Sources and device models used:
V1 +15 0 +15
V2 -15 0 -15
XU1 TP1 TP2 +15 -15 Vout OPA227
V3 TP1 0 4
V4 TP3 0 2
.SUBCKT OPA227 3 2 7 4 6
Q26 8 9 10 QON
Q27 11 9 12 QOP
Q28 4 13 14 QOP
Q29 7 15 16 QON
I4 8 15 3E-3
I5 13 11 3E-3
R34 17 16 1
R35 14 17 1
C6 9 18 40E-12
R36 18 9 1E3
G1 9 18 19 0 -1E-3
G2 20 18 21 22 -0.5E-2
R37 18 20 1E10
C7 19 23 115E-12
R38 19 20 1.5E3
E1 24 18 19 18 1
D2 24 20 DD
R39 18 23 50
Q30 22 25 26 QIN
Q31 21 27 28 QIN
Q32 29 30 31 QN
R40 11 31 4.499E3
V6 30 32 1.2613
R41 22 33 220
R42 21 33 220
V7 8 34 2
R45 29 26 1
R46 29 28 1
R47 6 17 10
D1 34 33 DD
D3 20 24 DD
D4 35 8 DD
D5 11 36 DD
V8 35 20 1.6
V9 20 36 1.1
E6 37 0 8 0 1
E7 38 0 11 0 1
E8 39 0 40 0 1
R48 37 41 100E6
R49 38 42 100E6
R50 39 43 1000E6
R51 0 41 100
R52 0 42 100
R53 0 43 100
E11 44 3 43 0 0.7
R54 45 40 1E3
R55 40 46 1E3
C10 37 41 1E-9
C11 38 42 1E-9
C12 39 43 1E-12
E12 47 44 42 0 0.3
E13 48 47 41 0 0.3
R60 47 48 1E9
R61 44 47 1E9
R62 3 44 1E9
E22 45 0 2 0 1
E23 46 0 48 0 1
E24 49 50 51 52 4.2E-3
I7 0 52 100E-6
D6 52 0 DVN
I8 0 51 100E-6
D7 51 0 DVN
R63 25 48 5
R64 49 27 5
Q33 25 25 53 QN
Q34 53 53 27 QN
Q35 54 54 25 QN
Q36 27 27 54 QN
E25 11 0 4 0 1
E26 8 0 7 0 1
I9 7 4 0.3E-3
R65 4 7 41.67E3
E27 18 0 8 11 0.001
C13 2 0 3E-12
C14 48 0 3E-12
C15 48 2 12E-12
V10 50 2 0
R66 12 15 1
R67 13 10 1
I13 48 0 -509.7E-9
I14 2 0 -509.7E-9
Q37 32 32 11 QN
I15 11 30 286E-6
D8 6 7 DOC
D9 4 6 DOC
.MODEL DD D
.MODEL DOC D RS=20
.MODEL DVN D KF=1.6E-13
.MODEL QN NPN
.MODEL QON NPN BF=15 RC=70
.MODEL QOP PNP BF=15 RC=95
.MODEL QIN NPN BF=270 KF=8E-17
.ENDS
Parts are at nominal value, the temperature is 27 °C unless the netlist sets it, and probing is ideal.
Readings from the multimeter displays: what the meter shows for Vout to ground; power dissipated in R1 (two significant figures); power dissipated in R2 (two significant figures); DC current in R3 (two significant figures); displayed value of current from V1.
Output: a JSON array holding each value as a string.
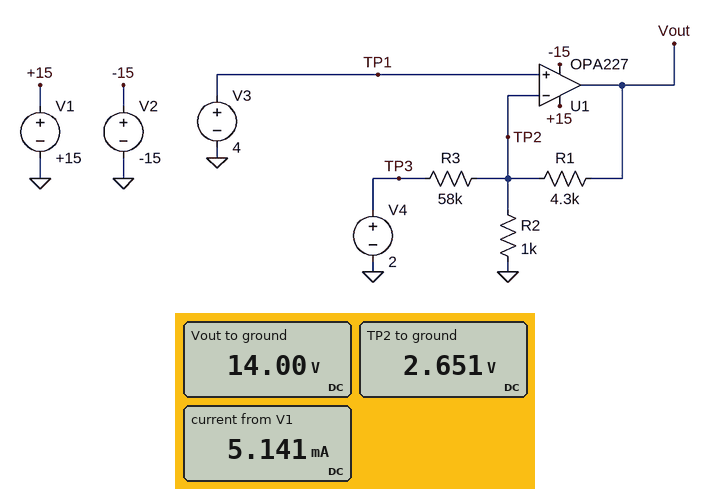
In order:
["14.00 V", "30 mW", "7.0 mW", "11 µA", "5.141 mA"]
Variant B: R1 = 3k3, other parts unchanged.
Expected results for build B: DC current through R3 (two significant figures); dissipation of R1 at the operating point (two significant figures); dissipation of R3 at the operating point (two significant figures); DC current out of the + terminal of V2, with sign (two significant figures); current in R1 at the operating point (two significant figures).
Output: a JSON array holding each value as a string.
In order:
["21 µA", "35 mW", "26 µW", "-2.5 mA", "3.3 mA"]
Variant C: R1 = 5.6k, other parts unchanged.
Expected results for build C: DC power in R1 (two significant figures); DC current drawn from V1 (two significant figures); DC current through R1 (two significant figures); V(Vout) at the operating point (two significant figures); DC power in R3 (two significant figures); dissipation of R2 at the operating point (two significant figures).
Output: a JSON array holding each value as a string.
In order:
["24 mW", "4.8 mA", "2.1 mA", "14 V", "4.1 µW", "6.2 mW"]
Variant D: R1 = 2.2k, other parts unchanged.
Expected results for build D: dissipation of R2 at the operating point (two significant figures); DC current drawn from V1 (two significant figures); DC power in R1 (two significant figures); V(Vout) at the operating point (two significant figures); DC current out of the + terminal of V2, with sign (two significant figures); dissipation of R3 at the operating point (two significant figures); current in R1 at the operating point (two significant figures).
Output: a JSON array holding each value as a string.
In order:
["16 mW", "6.1 mA", "36 mW", "13 V", "-2.3 mA", "69 µW", "4.0 mA"]
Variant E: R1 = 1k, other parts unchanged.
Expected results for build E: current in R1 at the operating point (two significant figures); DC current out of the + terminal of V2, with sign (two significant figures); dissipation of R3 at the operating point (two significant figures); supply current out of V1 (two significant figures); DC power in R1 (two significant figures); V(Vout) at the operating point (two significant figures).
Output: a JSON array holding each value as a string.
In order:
["4.0 mA", "-2.3 mA", "69 µW", "6.1 mA", "16 mW", "8.0 V"]
